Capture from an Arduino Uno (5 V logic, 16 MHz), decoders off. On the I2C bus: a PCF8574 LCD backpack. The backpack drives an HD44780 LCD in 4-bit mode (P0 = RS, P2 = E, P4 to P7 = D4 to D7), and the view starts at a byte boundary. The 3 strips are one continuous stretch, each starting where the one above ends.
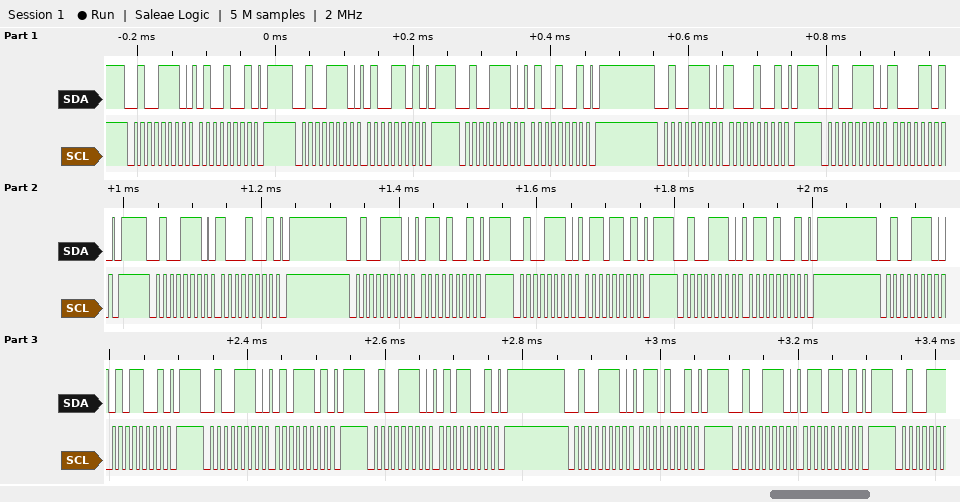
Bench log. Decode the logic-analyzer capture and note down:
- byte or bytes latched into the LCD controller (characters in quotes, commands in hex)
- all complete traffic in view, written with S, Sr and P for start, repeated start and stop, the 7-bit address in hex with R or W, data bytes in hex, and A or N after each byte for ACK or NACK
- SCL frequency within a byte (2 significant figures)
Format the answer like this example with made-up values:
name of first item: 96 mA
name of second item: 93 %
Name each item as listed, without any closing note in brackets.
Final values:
byte or bytes latched into the LCD controller: 'H' 'e'
all complete traffic in view, written with S, Sr and P for start, repeated start and stop, the 7-bit address in hex with R or W, data bytes in hex, and A or N after each byte for ACK or NACK: S 27W A 49 A P S 27W A 4D A P S 27W A 49 A P S 27W A 89 A P S 27W A 8D A P S 27W A 89 A P S 27W A 69 A P S 27W A 6D A P S 27W A 69 A P S 27W A 59 A P S 27W A 5D A P S 27W A 59 A P S 27W A 69 A P S 27W A 6D A P
SCL frequency within a byte: 100 kHz
